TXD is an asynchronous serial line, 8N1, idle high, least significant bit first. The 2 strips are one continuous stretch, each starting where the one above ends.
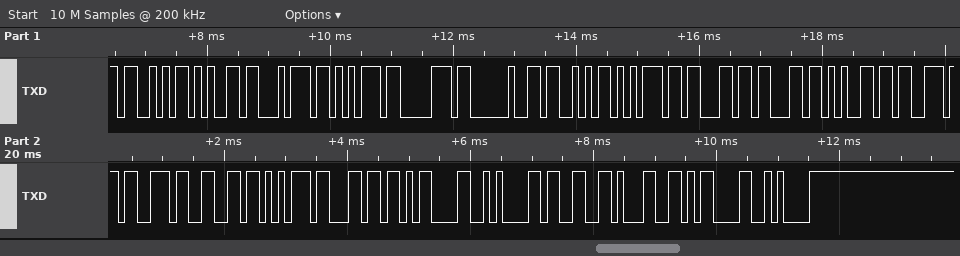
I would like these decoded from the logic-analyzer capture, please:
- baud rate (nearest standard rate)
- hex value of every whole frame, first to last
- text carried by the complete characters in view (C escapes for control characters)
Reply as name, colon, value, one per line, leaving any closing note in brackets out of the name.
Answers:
baud rate: 9600 baud
hex value of every whole frame, first to last: 0x53 0x65 0x74 0x75 0x70 0x20 0x53 0x75 0x63 0x63 0x65 0x73 0x73 0x66 0x75 0x6C 0x0D 0x0A 0x33 0x31 0x0D 0x0A
text carried by the complete characters in view: "Setup Successful\r\n31\r\n"
